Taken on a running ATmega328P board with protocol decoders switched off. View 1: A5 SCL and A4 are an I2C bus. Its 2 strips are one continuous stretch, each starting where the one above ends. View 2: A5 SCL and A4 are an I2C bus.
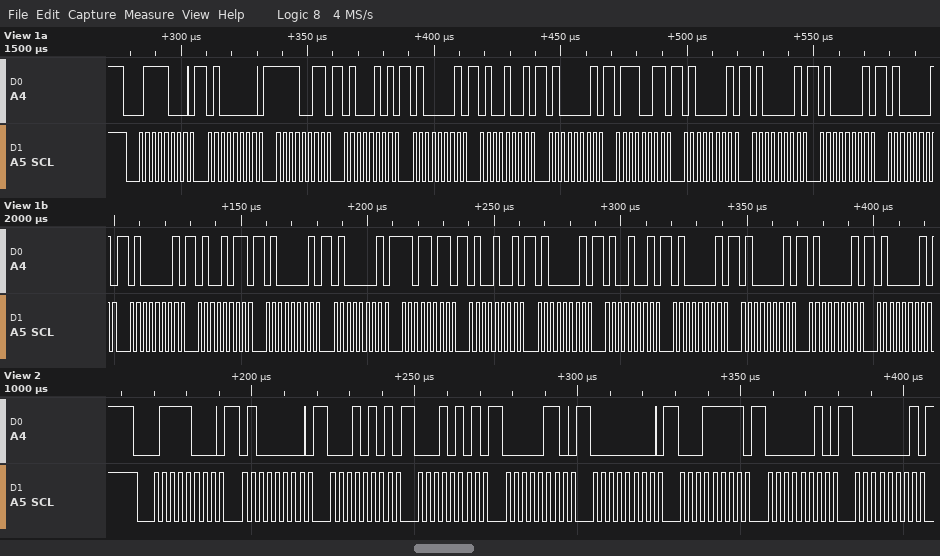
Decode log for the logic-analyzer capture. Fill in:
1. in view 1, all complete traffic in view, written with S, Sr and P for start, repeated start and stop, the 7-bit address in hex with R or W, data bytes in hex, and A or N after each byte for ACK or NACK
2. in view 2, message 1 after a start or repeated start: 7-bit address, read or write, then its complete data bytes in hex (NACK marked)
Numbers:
S 3CW A 40 A F3 A 45 A 41 A 49 A 41 A 73 A 41 A 41 A 41 A 41 A 41 A 4B A 41 A 41 A DB A 49 A 41 A 49 A 41 A 41 A 41 A 41 A
0x3C write: 40 15 15 06 00 1F 02 01
